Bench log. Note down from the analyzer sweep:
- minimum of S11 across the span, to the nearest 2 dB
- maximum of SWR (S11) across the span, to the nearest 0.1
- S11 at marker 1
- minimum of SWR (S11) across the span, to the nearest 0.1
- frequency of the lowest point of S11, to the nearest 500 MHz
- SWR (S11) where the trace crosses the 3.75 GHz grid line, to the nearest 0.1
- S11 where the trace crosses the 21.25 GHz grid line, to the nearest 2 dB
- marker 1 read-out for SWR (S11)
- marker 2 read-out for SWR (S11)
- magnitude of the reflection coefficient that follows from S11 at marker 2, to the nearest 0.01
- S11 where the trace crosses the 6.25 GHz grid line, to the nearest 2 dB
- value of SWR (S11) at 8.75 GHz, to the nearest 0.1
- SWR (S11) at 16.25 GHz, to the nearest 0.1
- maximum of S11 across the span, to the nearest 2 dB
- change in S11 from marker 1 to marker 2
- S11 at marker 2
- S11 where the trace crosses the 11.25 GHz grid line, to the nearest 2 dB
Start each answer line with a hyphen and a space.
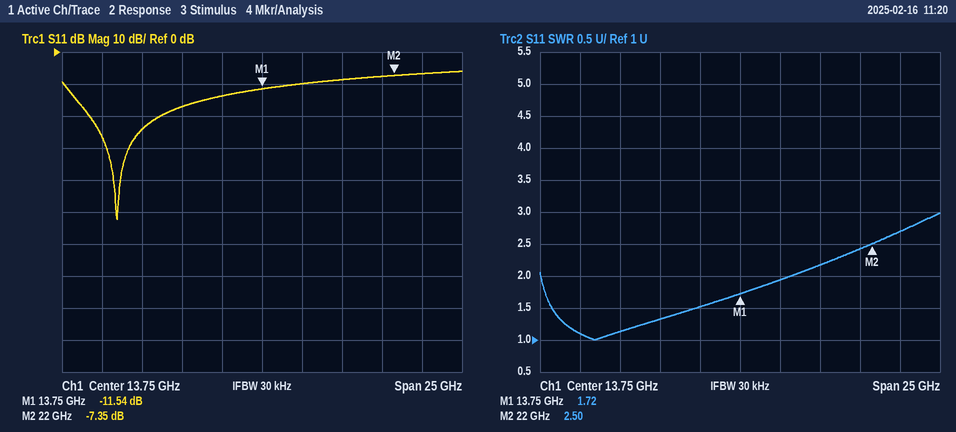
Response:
- -52 dB
- 3.0
- -11.54 dB
- 1.0
- 4.5 GHz
- 1.1
- -8 dB
- 1.72
- 2.50
- 0.43
- -24 dB
- 1.3
- 1.9
- -6 dB
- 4.19 dB
- -7.35 dB
- -14 dB
